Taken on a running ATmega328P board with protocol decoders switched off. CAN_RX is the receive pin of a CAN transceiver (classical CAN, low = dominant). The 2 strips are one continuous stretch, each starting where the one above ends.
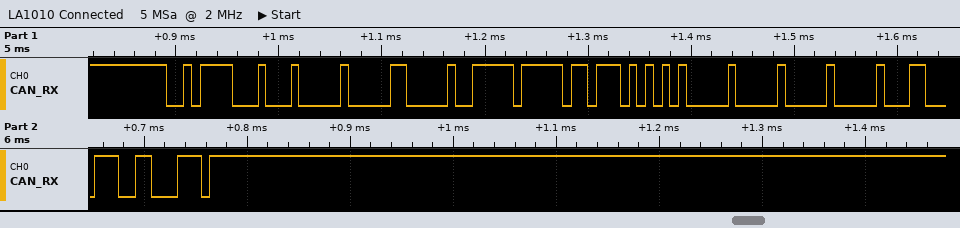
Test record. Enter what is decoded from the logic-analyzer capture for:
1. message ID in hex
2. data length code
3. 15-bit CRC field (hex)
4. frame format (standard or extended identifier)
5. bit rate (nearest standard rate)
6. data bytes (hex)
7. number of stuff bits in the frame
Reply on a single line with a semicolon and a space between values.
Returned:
0x2F1; 8; 0x0E63; standard; 125 kbit/s; 01 01 FF EE AA 00 00 03; 9
